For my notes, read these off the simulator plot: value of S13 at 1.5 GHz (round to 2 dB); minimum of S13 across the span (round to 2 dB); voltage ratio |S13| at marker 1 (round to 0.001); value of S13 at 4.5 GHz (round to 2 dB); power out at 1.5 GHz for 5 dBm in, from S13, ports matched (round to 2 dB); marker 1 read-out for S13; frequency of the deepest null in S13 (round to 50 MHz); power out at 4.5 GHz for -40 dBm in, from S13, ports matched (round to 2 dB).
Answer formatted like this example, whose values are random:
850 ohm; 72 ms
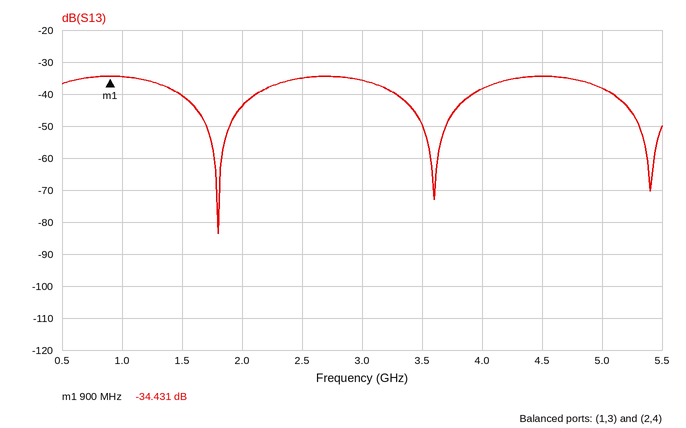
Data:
-40 dB; -84 dB; 0.019; -34 dB; -36 dBm; -34.431 dB; 1.80 GHz; -74 dBm
